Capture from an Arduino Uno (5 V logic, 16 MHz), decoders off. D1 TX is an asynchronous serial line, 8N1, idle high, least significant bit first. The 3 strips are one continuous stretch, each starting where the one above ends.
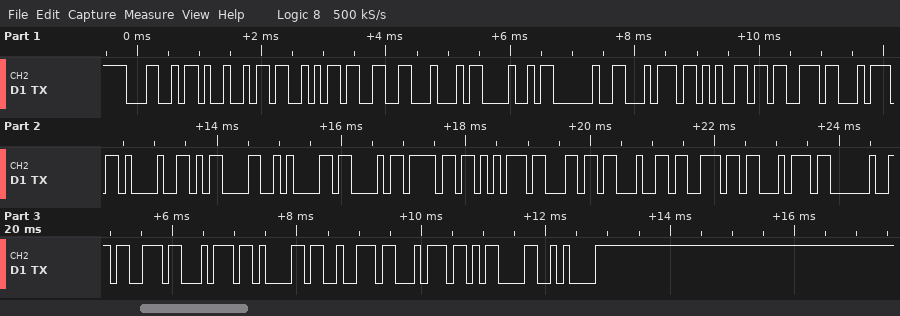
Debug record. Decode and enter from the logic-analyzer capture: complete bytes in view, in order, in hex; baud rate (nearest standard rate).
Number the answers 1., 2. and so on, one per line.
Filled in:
1. 4C 49 53 33 44 48 20 74 65 73 74 21 0D 0A 43 6F 75 6C 64 6E 74 20 73 74 61 72 74 0D 0A
2. 9600 baud
